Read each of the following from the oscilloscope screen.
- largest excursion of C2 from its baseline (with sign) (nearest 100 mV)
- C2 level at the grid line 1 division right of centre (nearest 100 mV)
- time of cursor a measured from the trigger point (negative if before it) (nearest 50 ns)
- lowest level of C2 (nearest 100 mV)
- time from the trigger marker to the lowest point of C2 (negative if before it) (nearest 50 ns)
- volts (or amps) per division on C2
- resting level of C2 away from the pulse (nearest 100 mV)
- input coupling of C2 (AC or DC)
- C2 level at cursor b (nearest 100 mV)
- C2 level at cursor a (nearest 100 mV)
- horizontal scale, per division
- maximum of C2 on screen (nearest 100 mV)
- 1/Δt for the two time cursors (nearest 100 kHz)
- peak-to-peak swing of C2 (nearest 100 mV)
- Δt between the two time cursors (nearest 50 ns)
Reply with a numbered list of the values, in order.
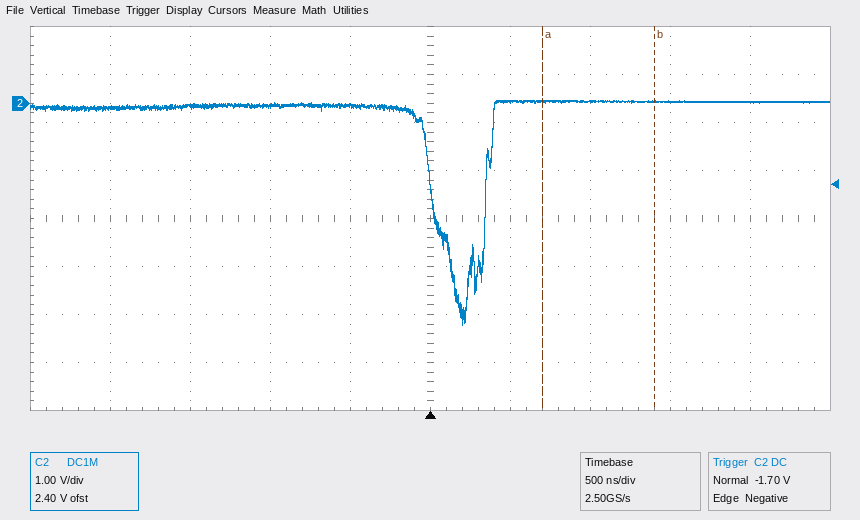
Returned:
1. -4.6 V
2. 0.0 V
3. +700 ns
4. -4.6 V
5. +200 ns
6. 1 V
7. 0.0 V
8. DC
9. 0.0 V
10. 0.0 V
11. 500 ns
12. 100 mV
13. 1.4 MHz
14. 4.7 V
15. 700 ns
